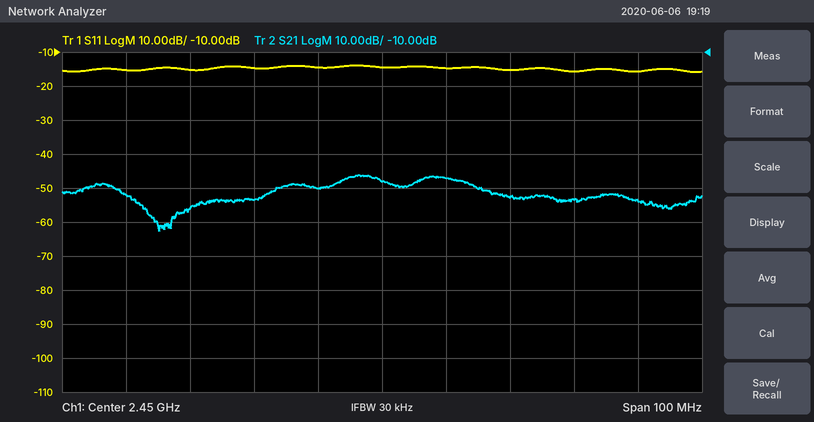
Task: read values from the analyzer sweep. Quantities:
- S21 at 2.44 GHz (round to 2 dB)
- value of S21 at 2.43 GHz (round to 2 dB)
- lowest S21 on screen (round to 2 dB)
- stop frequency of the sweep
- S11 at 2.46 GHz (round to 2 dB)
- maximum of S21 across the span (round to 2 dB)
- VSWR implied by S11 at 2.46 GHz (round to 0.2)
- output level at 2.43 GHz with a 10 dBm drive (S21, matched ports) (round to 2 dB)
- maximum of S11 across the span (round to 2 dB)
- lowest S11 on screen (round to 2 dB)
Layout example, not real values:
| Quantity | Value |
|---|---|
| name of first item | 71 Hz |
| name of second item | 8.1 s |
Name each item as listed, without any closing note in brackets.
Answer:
| Quantity | Value |
|---|---|
| S21 at 2.44 GHz | -50 dB |
| value of S21 at 2.43 GHz | -54 dB |
| lowest S21 on screen | -62 dB |
| stop frequency of the sweep | 2.5 GHz |
| S11 at 2.46 GHz | -14 dB |
| maximum of S21 across the span | -46 dB |
| VSWR implied by S11 at 2.46 GHz | 1.4 |
| output level at 2.43 GHz with a 10 dBm drive (S21, matched ports) | -44 dBm |
| maximum of S11 across the span | -14 dB |
| lowest S11 on screen | -16 dB |
